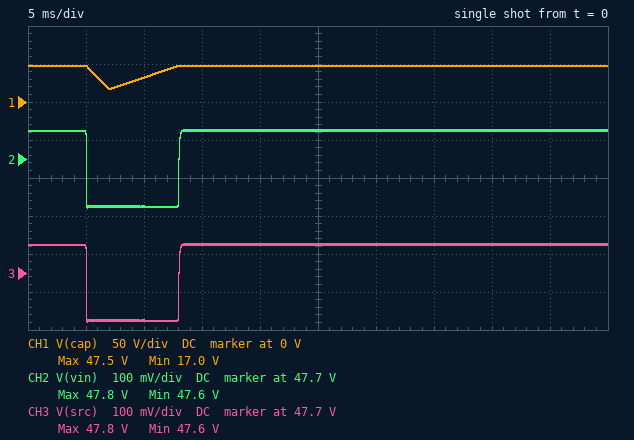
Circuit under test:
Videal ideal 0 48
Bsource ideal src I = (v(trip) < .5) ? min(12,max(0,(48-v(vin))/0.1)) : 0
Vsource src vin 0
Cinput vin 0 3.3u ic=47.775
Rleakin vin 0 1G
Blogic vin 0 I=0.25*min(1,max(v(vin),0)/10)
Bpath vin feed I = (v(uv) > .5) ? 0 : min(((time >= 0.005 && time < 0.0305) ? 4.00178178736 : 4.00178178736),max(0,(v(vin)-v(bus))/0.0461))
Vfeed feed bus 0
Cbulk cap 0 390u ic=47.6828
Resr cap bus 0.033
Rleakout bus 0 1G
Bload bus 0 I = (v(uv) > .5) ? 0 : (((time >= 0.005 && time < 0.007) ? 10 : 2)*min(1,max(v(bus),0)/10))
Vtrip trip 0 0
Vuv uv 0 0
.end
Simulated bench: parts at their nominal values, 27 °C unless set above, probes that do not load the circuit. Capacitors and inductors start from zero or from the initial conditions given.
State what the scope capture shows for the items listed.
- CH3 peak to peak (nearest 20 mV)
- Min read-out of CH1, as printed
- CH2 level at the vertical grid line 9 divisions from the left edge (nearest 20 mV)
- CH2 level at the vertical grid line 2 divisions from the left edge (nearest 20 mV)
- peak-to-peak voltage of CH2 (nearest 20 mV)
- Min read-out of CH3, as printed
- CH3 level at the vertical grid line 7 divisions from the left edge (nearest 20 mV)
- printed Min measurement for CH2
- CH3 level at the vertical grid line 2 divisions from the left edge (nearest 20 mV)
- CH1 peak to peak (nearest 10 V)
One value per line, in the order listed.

200 mV
17.0 V
47.78 V
47.58 V
200 mV
47.6 V
47.78 V
47.6 V
47.58 V
30 V
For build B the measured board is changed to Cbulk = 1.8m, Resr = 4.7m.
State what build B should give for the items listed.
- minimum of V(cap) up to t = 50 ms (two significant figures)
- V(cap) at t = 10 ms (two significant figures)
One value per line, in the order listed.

41 V
44 V
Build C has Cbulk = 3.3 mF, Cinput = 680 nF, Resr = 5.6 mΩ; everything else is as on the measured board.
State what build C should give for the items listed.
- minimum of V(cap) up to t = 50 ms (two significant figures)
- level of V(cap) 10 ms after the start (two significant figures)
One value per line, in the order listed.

44 V
46 V
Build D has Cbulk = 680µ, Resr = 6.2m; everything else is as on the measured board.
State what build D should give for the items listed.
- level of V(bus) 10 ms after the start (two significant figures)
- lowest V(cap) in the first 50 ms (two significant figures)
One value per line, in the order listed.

39 V
30 V
